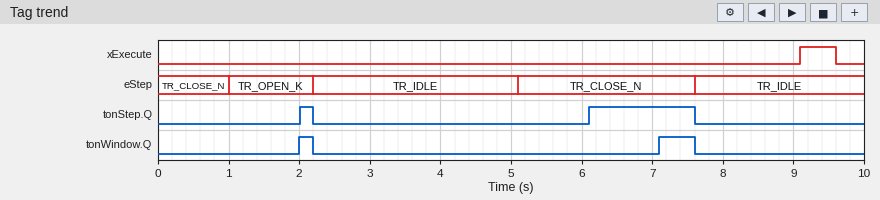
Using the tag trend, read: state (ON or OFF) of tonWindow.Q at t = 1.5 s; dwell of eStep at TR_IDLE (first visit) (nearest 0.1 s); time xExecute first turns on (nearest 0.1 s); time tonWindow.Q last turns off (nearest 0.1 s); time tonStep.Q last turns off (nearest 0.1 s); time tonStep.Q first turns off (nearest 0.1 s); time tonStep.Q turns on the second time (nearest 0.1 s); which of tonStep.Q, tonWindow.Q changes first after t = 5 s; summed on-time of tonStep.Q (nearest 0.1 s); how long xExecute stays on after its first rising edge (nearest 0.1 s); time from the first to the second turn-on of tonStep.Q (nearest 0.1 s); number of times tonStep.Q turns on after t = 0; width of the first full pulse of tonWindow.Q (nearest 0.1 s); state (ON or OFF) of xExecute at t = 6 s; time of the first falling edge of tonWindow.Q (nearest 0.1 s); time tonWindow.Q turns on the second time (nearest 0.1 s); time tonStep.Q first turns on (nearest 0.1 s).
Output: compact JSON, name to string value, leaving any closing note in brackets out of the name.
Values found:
{"state (ON or OFF) of tonWindow.Q at t = 1.5 s": "OFF", "dwell of eStep at TR_IDLE (first visit)": "2.9 s", "time xExecute first turns on": "9.1 s", "time tonWindow.Q last turns off": "7.6 s", "time tonStep.Q last turns off": "7.6 s", "time tonStep.Q first turns off": "2.2 s", "time tonStep.Q turns on the second time": "6.1 s", "which of tonStep.Q, tonWindow.Q changes first after t = 5 s": "tonStep.Q", "summed on-time of tonStep.Q": "1.7 s", "how long xExecute stays on after its first rising edge": "0.5 s", "time from the first to the second turn-on of tonStep.Q": "4.1 s", "number of times tonStep.Q turns on after t = 0": "2", "width of the first full pulse of tonWindow.Q": "0.2 s", "state (ON or OFF) of xExecute at t = 6 s": "OFF", "time of the first falling edge of tonWindow.Q": "2.2 s", "time tonWindow.Q turns on the second time": "7.1 s", "time tonStep.Q first turns on": "2.0 s"}
